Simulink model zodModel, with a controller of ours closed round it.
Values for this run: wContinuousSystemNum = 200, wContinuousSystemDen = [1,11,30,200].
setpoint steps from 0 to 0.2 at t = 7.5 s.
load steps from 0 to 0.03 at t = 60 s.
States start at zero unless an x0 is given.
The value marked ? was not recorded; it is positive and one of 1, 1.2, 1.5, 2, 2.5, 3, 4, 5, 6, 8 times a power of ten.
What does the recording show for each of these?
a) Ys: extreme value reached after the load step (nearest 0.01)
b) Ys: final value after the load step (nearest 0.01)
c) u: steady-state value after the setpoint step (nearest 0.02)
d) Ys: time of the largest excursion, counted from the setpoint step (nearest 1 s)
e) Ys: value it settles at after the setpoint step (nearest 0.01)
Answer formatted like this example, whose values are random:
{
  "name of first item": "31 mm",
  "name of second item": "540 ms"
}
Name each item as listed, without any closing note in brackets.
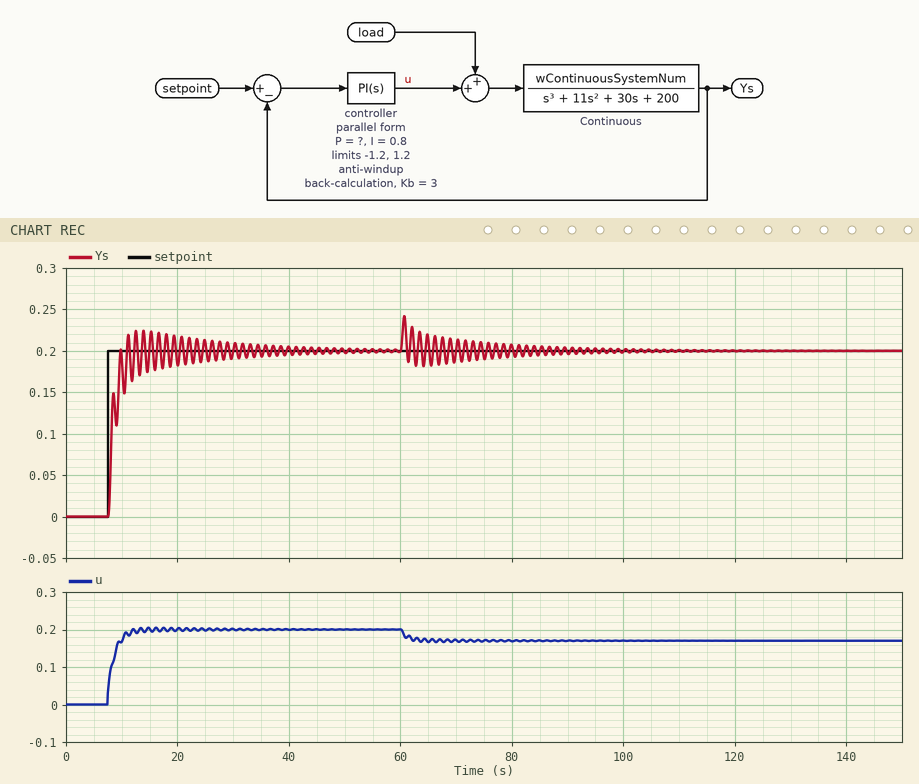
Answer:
{
  "Ys: extreme value reached after the load step": "0.24",
  "Ys: final value after the load step": "0.20",
  "u: steady-state value after the setpoint step": "0.20",
  "Ys: time of the largest excursion, counted from the setpoint step": "6 s",
  "Ys: value it settles at after the setpoint step": "0.20"
}
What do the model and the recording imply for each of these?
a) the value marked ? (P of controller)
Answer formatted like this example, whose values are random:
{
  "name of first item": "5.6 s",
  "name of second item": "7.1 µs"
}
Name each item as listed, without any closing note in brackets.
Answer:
{
  "the value marked ?": "0.15"
}
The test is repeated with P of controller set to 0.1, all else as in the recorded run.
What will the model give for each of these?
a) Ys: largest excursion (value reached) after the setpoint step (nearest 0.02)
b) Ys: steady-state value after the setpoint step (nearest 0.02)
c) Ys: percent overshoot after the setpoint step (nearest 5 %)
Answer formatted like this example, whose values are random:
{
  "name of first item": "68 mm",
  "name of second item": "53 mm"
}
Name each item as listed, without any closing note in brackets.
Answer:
{
  "Ys: largest excursion (value reached) after the setpoint step": "0.22",
  "Ys: steady-state value after the setpoint step": "0.20",
  "Ys: percent overshoot after the setpoint step": "10 %"
}
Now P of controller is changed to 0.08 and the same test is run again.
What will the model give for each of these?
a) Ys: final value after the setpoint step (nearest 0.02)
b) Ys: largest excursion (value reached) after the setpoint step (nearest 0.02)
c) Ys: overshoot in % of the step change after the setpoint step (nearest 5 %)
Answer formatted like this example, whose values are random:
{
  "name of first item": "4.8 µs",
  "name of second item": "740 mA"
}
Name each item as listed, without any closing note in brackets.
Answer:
{
  "Ys: final value after the setpoint step": "0.20",
  "Ys: largest excursion (value reached) after the setpoint step": "0.22",
  "Ys: overshoot in % of the step change after the setpoint step": "10 %"
}
